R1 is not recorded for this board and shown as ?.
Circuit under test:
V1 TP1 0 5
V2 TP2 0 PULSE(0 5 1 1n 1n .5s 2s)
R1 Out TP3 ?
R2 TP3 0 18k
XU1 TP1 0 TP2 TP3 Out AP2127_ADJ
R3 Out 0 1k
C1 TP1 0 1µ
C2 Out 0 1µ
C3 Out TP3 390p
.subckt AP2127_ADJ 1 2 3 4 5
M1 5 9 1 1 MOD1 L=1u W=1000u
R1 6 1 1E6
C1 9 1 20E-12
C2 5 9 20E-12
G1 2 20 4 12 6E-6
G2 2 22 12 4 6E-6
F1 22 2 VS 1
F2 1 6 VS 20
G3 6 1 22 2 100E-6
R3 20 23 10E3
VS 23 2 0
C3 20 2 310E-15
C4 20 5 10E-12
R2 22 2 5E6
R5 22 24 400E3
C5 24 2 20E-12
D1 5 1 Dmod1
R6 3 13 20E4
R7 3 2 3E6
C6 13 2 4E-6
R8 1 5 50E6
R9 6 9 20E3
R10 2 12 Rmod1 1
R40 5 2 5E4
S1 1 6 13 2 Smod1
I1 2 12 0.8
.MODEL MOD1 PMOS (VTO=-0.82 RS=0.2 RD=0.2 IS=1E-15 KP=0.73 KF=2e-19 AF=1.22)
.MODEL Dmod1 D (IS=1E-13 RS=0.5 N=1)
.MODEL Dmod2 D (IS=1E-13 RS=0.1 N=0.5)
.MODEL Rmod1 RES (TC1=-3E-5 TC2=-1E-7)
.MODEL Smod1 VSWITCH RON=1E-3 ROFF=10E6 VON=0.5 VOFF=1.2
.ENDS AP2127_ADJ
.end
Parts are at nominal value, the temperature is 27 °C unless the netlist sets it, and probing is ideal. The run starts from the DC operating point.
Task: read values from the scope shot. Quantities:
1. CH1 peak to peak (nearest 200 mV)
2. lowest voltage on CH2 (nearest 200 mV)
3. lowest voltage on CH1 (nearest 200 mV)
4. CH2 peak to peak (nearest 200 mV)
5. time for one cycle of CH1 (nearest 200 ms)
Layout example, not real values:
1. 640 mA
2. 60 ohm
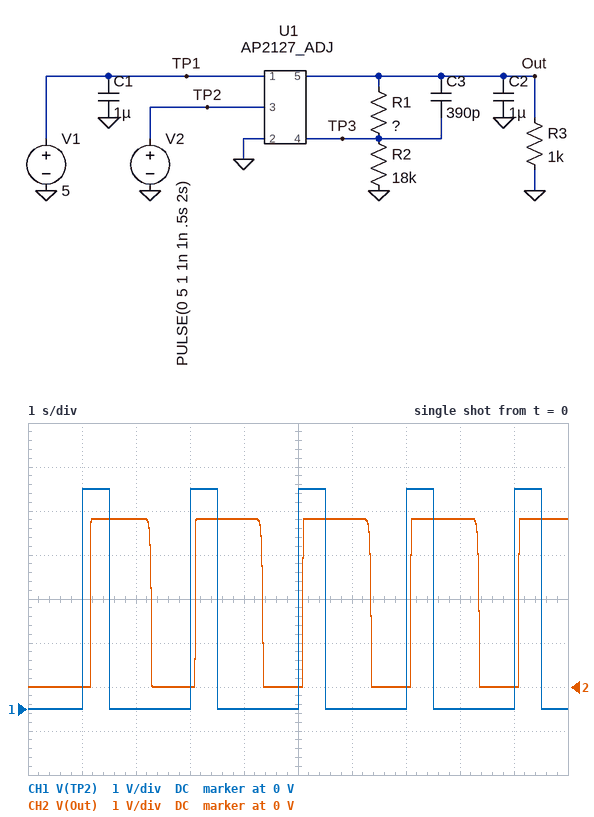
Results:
1. 5.0 V
2. 0 V
3. 0 V
4. 3.8 V
5. 2.0 s
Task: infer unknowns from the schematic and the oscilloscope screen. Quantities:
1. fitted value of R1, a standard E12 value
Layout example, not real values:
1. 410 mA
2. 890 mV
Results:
1. 68 kΩ
